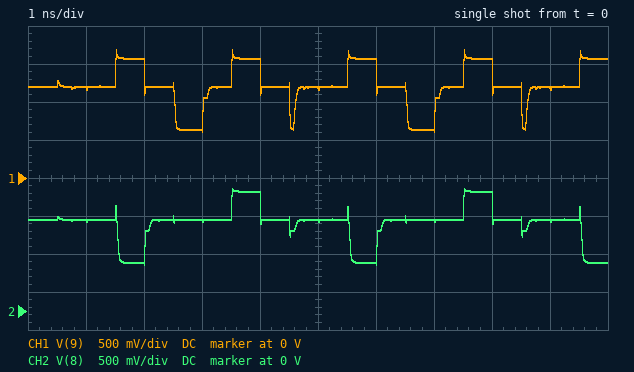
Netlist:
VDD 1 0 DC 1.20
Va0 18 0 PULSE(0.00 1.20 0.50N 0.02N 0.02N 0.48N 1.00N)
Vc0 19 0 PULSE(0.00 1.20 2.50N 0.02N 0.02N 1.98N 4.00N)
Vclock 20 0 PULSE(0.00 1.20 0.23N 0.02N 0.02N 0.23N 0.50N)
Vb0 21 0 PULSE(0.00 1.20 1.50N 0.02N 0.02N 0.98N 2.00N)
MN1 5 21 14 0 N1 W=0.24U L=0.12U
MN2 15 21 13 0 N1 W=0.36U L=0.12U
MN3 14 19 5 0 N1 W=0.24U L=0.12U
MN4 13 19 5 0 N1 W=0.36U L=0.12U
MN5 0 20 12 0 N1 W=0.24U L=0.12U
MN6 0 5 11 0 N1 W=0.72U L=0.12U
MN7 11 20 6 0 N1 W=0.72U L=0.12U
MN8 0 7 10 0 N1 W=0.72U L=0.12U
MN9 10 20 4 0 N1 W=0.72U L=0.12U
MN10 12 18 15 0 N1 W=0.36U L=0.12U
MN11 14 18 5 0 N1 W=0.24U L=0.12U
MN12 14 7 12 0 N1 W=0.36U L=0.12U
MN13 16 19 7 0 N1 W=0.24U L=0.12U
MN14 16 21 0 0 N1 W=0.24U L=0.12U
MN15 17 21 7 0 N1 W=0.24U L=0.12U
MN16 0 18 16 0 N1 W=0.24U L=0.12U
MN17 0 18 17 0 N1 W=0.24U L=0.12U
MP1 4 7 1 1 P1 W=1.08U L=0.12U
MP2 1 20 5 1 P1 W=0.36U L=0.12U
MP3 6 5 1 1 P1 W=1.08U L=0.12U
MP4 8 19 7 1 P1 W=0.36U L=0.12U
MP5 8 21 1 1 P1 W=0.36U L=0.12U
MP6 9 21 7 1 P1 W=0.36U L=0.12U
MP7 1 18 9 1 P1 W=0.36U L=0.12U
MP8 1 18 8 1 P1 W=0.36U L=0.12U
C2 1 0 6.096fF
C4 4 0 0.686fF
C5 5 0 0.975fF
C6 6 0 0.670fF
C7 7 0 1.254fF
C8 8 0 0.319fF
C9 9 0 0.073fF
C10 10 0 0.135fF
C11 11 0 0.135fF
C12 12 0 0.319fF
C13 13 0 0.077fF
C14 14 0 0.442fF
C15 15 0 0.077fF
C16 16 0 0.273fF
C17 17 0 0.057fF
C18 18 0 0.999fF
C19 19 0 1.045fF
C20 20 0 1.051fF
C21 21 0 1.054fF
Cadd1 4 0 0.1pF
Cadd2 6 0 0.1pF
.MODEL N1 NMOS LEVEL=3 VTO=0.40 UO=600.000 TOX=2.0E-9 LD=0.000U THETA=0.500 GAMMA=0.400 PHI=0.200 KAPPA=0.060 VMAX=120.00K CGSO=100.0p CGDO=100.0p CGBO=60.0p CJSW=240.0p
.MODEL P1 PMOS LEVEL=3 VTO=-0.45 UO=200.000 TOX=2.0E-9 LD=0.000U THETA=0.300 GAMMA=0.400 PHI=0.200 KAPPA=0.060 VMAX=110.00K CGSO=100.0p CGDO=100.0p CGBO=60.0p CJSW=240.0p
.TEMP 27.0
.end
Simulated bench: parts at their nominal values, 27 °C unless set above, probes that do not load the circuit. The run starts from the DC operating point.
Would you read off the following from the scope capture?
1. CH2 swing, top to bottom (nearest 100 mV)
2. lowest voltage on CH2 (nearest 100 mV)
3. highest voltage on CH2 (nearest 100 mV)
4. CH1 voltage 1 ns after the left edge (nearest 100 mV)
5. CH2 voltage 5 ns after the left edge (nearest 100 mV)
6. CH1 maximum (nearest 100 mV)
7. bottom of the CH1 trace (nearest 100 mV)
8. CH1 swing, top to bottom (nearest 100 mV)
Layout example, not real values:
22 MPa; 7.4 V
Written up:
1.0 V; 600 mV; 1.6 V; 1.2 V; 1.2 V; 1.7 V; 600 mV; 1.1 V
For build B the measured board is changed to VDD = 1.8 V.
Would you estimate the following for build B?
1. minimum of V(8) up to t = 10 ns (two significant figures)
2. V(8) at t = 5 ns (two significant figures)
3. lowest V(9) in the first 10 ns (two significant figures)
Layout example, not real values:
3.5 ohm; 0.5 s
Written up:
900 mV; 1.8 V; 840 mV
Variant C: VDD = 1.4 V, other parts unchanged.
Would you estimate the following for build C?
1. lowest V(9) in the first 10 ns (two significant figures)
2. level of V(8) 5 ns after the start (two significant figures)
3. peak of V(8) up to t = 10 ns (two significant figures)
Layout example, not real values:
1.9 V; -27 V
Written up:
650 mV; 1.4 V; 1.7 V
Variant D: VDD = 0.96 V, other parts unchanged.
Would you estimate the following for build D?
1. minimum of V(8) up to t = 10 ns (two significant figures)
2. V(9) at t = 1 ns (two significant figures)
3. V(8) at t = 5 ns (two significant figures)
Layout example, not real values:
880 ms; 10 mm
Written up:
550 mV; 960 mV; 950 mV
